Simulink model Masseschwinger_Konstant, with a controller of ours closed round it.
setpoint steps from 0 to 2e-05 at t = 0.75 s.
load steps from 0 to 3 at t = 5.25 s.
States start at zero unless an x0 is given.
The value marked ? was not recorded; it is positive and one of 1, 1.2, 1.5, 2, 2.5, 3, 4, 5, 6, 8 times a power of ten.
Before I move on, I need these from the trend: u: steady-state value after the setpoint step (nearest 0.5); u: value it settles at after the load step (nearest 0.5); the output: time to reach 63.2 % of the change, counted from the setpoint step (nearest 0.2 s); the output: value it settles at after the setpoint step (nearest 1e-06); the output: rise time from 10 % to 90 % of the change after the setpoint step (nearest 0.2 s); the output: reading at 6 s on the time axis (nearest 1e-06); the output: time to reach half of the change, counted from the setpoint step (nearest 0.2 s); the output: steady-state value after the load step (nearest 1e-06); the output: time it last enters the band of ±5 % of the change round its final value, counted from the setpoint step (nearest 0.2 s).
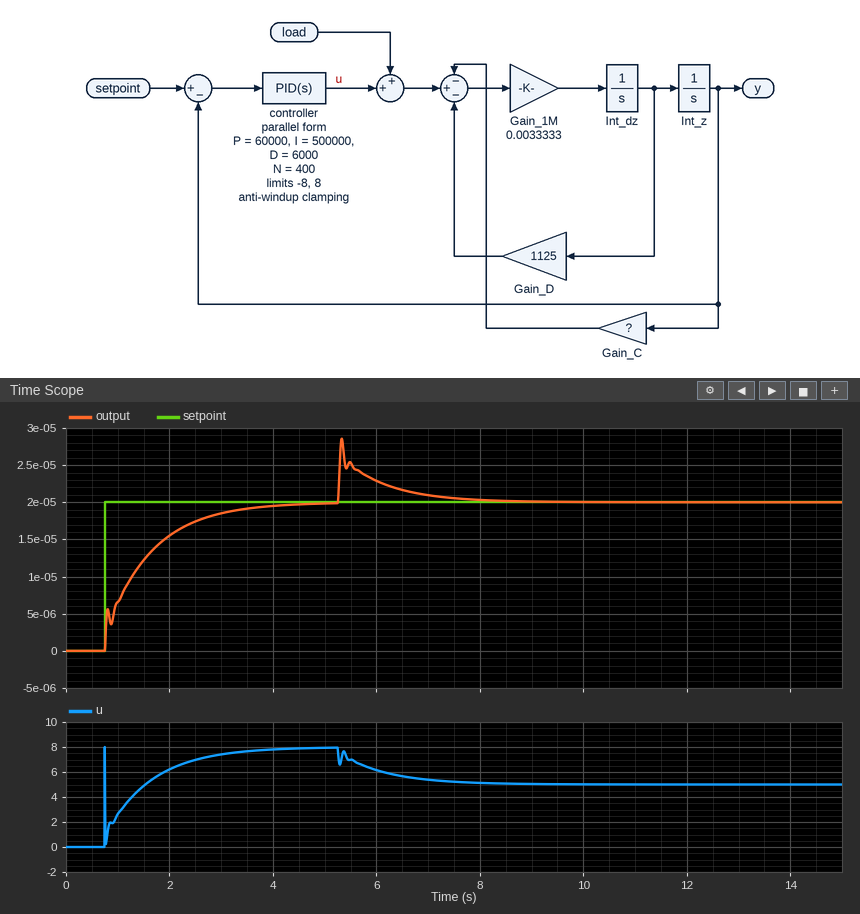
8.0
5.0
0.8 s
0.000020
2.0 s
0.000023
0.6 s
0.000020
2.6 s
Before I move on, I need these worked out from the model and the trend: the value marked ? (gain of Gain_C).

400000
